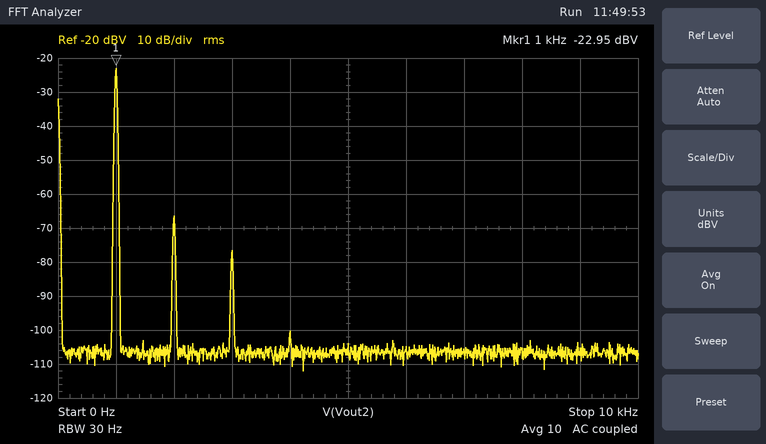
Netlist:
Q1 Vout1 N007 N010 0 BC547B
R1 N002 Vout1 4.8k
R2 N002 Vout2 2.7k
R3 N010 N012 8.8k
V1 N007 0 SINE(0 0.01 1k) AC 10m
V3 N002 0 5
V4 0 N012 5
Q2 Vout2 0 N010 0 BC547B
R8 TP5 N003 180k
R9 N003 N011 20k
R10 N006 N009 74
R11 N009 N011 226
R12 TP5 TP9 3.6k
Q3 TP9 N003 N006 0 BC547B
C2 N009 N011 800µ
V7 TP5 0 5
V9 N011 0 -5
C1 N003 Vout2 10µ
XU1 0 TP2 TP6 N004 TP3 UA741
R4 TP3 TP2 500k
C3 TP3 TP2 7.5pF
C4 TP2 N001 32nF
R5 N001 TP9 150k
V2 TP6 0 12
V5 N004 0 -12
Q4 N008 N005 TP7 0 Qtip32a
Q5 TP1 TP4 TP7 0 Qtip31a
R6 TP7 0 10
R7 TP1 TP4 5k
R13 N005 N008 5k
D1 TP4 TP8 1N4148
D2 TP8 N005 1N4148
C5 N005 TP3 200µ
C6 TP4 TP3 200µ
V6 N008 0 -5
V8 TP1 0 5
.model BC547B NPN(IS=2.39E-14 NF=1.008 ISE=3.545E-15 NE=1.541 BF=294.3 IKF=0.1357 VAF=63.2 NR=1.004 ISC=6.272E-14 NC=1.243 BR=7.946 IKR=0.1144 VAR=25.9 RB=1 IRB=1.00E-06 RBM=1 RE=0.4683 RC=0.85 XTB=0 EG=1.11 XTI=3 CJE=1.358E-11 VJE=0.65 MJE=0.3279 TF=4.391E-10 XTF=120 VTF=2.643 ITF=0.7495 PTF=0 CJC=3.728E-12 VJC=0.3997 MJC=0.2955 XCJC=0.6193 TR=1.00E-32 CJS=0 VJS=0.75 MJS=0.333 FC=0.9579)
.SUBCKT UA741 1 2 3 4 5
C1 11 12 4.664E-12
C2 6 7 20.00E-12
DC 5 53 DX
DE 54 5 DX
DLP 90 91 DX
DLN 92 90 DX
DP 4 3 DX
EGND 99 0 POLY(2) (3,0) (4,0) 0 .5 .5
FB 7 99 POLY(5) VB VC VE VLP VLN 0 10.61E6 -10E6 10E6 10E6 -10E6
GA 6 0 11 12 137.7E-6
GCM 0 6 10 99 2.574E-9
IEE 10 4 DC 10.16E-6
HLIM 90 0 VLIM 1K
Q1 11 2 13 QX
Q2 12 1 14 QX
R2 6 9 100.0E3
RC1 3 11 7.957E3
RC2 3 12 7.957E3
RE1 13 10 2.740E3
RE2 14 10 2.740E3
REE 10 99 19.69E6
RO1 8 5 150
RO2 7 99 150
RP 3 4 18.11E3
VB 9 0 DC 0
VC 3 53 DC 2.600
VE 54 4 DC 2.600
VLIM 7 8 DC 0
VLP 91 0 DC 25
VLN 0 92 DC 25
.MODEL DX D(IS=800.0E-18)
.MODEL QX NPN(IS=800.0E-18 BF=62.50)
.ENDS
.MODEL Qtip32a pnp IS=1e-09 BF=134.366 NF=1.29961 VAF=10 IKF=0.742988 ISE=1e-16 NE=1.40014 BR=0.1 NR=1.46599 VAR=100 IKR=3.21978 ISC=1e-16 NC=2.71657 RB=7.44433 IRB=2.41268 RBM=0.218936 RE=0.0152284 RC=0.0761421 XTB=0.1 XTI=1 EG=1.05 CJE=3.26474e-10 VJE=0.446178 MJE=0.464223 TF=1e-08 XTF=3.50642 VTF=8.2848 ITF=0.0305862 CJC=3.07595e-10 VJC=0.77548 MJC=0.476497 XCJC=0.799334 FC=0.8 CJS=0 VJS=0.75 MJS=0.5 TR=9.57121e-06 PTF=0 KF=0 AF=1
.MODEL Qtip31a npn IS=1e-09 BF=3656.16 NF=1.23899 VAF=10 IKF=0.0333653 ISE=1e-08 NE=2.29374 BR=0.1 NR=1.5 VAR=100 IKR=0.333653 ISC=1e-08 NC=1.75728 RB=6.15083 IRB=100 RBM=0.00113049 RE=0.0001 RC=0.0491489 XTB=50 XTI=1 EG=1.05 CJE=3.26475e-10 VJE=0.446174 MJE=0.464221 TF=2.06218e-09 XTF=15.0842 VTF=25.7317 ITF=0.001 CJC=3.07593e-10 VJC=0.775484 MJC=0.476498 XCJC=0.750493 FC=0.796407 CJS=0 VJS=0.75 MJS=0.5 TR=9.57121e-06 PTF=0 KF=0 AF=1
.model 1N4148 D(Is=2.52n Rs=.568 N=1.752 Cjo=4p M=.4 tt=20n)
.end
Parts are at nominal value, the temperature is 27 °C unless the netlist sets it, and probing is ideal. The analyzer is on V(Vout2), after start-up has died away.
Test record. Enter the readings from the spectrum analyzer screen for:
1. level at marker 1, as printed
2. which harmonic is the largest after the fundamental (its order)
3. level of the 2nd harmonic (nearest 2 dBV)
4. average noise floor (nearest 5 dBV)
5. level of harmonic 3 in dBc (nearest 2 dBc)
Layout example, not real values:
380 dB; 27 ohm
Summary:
-22.95 dBV; 2; -66 dBV; -105 dBV; -54 dBc
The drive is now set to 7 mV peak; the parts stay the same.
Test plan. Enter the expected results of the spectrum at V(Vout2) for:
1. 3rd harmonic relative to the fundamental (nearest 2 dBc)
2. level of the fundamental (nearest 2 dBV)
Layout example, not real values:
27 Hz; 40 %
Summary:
-60 dBc; -26 dBV
